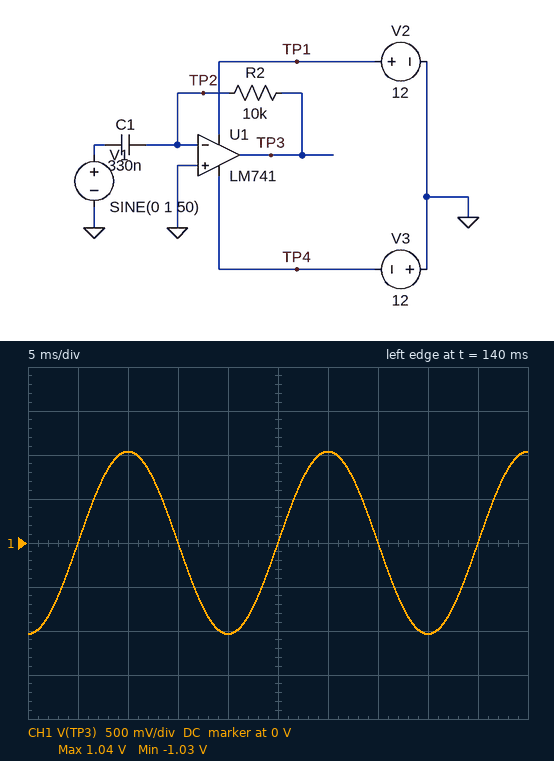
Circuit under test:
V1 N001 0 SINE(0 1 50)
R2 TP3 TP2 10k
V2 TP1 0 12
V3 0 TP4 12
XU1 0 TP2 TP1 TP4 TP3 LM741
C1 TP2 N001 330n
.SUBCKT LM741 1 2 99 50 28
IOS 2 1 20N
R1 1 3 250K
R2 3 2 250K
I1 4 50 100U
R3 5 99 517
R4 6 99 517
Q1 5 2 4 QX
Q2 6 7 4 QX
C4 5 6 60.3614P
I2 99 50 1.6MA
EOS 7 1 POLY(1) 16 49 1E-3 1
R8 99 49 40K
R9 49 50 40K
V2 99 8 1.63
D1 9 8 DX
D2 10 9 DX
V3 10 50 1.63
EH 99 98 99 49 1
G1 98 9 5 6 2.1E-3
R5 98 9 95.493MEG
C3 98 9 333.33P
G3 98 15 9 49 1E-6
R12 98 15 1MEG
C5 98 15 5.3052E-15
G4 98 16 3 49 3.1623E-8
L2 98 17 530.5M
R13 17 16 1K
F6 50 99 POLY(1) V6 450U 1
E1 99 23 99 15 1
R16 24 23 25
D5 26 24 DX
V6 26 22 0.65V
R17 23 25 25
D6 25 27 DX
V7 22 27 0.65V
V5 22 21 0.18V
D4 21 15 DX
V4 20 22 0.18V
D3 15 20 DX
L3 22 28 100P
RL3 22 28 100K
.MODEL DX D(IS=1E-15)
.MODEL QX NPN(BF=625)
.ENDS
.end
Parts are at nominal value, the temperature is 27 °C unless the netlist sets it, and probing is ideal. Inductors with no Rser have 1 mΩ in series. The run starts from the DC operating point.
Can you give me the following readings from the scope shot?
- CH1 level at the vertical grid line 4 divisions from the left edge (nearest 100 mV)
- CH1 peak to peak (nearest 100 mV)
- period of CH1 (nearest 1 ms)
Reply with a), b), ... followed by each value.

a) -1.0 V
b) 2.1 V
c) 20 ms
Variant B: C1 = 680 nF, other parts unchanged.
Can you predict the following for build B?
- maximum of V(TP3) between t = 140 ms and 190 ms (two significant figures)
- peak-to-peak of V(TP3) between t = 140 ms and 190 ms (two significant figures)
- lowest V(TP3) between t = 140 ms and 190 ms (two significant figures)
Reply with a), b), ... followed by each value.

a) 2.1 V
b) 4.3 V
c) -2.1 V
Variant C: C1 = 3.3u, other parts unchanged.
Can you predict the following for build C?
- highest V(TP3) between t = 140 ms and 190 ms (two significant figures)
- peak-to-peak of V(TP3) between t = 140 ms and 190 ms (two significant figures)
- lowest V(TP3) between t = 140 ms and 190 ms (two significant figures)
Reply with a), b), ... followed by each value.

a) 10 V
b) 21 V
c) -10 V
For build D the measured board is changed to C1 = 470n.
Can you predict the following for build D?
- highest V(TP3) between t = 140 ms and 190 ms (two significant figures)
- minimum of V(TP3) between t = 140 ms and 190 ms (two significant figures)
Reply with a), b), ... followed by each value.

a) 1.5 V
b) -1.5 V
